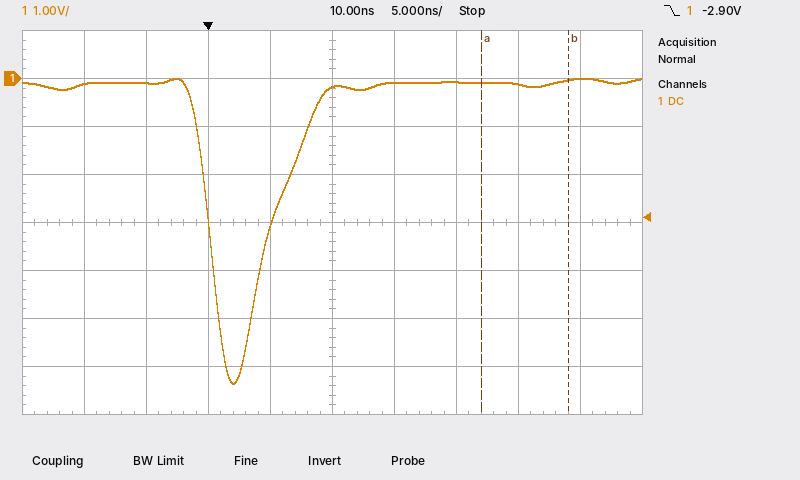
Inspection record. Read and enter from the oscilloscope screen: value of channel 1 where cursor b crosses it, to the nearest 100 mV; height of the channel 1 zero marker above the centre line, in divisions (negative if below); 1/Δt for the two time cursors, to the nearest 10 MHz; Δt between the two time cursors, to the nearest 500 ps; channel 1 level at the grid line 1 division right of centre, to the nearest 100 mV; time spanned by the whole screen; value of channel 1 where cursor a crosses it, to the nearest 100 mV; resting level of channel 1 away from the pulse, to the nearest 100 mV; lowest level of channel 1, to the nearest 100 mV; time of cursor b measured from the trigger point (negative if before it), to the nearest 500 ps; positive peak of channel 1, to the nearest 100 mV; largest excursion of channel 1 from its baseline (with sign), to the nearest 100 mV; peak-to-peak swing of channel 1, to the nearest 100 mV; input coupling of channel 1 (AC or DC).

0.0 V
+3.0 div
140 MHz
7.0 ns
-100 mV
50 ns
-100 mV
-100 mV
-6.4 V
+29.0 ns
0.0 V
-6.3 V
6.4 V
DC
